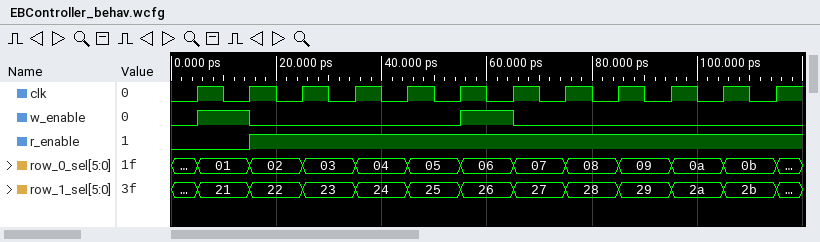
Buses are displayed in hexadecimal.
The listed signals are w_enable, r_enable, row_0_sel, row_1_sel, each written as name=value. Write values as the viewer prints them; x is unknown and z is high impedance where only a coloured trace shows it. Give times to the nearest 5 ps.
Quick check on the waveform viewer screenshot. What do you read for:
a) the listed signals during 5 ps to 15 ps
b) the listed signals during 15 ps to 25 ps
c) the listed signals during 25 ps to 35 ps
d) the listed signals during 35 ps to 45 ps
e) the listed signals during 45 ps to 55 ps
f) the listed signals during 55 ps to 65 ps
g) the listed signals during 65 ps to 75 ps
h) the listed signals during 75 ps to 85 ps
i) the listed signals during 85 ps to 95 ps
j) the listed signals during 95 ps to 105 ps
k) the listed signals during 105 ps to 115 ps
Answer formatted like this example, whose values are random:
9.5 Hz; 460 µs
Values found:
w_enable=1, r_enable=0, row_0_sel=01, row_1_sel=21; w_enable=0, r_enable=1, row_0_sel=02, row_1_sel=22; w_enable=0, r_enable=1, row_0_sel=03, row_1_sel=23; w_enable=0, r_enable=1, row_0_sel=04, row_1_sel=24; w_enable=0, r_enable=1, row_0_sel=05, row_1_sel=25; w_enable=1, r_enable=1, row_0_sel=06, row_1_sel=26; w_enable=0, r_enable=1, row_0_sel=07, row_1_sel=27; w_enable=0, r_enable=1, row_0_sel=08, row_1_sel=28; w_enable=0, r_enable=1, row_0_sel=09, row_1_sel=29; w_enable=0, r_enable=1, row_0_sel=0a, row_1_sel=2a; w_enable=0, r_enable=1, row_0_sel=0b, row_1_sel=2b
